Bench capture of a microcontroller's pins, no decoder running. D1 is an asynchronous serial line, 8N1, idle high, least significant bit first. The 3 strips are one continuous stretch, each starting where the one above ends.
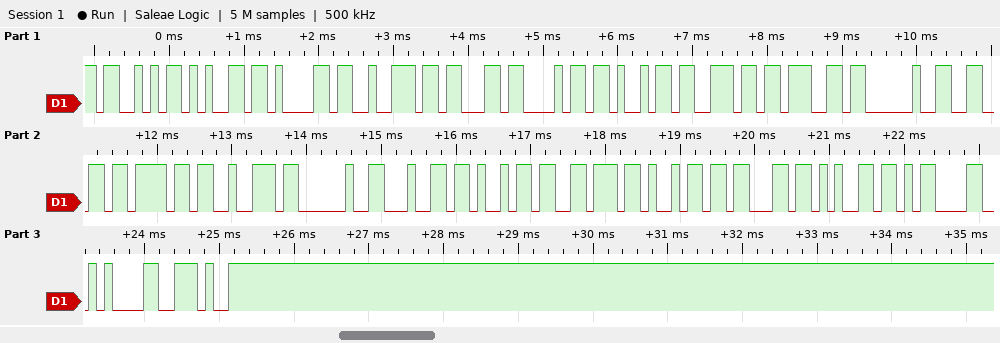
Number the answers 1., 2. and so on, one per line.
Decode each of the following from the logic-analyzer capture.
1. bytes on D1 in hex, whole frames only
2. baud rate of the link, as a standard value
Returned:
1. 53 65 61 72 63 68 69 6E 67 20 66 6F 72 20 64 69 76 69 63 65 0D 0A 2E
2. 9600 baud
